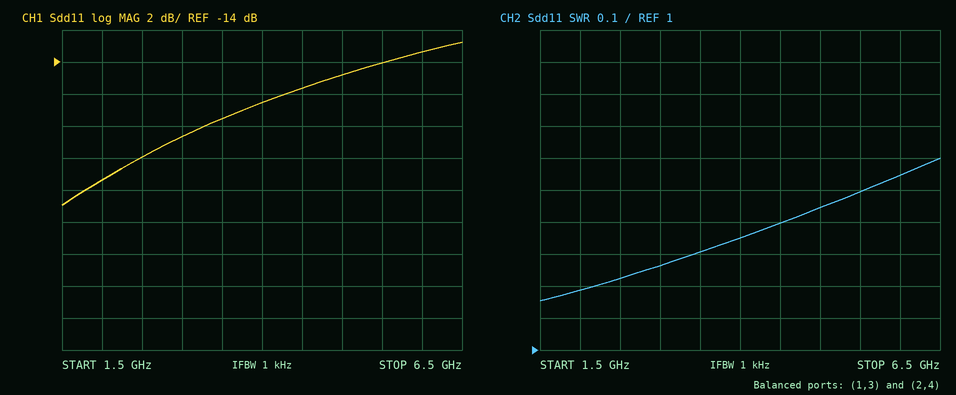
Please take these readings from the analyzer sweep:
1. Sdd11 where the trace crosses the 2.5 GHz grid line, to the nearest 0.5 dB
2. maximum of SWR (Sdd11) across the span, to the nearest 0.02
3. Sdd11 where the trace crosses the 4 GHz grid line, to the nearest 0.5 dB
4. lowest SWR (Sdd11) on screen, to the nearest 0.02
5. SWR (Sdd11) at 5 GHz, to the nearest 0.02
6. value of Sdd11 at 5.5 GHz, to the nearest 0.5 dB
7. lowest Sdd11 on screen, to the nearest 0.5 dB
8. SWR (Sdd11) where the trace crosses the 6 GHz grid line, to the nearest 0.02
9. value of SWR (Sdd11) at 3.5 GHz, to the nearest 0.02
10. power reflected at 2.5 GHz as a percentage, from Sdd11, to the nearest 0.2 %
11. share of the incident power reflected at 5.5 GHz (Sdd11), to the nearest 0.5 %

-20.0 dB
1.60
-16.5 dB
1.16
1.44
-14.0 dB
-23.0 dB
1.54
1.30
1.0 %
4.0 %
